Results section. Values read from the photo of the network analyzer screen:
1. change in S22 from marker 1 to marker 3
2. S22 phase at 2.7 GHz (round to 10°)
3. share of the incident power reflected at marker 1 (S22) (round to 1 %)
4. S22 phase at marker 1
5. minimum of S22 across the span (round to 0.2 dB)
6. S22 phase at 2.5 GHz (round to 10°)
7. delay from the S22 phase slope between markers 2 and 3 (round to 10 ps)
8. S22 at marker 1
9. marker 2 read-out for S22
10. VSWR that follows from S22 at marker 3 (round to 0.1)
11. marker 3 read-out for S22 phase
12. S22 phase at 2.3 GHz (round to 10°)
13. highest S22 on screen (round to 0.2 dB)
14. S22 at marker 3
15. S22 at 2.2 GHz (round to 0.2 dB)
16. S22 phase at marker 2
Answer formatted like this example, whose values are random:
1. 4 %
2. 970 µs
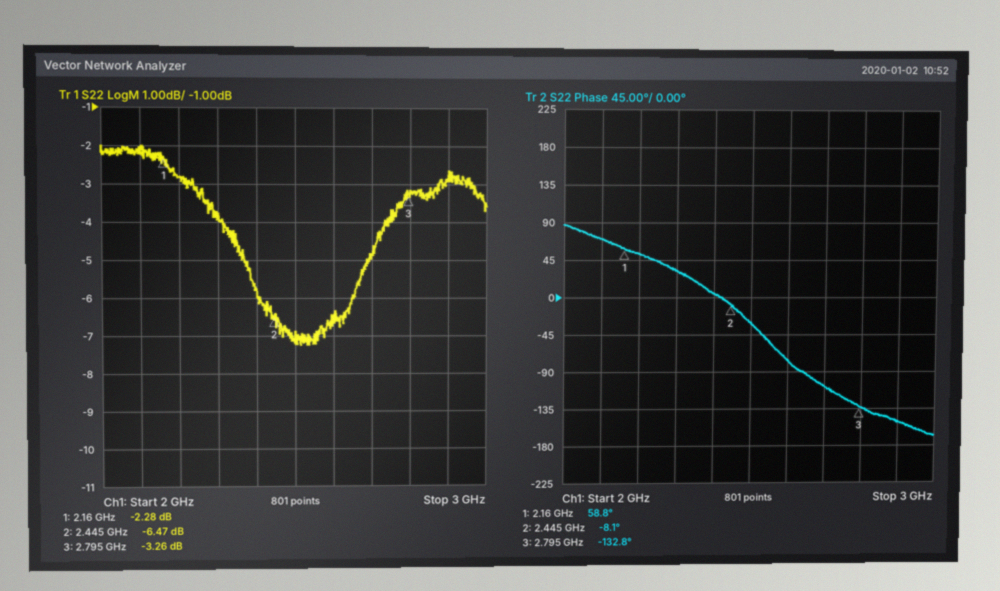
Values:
1. -0.98 dB
2. -110°
3. 59 %
4. 58.8°
5. -7.2 dB
6. -30°
7. 990 ps
8. -2.28 dB
9. -6.47 dB
10. 5.4
11. -132.8°
12. 30°
13. -2.0 dB
14. -3.26 dB
15. -2.8 dB
16. -8.1°
